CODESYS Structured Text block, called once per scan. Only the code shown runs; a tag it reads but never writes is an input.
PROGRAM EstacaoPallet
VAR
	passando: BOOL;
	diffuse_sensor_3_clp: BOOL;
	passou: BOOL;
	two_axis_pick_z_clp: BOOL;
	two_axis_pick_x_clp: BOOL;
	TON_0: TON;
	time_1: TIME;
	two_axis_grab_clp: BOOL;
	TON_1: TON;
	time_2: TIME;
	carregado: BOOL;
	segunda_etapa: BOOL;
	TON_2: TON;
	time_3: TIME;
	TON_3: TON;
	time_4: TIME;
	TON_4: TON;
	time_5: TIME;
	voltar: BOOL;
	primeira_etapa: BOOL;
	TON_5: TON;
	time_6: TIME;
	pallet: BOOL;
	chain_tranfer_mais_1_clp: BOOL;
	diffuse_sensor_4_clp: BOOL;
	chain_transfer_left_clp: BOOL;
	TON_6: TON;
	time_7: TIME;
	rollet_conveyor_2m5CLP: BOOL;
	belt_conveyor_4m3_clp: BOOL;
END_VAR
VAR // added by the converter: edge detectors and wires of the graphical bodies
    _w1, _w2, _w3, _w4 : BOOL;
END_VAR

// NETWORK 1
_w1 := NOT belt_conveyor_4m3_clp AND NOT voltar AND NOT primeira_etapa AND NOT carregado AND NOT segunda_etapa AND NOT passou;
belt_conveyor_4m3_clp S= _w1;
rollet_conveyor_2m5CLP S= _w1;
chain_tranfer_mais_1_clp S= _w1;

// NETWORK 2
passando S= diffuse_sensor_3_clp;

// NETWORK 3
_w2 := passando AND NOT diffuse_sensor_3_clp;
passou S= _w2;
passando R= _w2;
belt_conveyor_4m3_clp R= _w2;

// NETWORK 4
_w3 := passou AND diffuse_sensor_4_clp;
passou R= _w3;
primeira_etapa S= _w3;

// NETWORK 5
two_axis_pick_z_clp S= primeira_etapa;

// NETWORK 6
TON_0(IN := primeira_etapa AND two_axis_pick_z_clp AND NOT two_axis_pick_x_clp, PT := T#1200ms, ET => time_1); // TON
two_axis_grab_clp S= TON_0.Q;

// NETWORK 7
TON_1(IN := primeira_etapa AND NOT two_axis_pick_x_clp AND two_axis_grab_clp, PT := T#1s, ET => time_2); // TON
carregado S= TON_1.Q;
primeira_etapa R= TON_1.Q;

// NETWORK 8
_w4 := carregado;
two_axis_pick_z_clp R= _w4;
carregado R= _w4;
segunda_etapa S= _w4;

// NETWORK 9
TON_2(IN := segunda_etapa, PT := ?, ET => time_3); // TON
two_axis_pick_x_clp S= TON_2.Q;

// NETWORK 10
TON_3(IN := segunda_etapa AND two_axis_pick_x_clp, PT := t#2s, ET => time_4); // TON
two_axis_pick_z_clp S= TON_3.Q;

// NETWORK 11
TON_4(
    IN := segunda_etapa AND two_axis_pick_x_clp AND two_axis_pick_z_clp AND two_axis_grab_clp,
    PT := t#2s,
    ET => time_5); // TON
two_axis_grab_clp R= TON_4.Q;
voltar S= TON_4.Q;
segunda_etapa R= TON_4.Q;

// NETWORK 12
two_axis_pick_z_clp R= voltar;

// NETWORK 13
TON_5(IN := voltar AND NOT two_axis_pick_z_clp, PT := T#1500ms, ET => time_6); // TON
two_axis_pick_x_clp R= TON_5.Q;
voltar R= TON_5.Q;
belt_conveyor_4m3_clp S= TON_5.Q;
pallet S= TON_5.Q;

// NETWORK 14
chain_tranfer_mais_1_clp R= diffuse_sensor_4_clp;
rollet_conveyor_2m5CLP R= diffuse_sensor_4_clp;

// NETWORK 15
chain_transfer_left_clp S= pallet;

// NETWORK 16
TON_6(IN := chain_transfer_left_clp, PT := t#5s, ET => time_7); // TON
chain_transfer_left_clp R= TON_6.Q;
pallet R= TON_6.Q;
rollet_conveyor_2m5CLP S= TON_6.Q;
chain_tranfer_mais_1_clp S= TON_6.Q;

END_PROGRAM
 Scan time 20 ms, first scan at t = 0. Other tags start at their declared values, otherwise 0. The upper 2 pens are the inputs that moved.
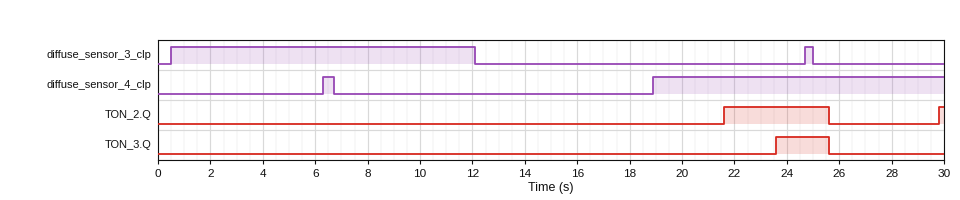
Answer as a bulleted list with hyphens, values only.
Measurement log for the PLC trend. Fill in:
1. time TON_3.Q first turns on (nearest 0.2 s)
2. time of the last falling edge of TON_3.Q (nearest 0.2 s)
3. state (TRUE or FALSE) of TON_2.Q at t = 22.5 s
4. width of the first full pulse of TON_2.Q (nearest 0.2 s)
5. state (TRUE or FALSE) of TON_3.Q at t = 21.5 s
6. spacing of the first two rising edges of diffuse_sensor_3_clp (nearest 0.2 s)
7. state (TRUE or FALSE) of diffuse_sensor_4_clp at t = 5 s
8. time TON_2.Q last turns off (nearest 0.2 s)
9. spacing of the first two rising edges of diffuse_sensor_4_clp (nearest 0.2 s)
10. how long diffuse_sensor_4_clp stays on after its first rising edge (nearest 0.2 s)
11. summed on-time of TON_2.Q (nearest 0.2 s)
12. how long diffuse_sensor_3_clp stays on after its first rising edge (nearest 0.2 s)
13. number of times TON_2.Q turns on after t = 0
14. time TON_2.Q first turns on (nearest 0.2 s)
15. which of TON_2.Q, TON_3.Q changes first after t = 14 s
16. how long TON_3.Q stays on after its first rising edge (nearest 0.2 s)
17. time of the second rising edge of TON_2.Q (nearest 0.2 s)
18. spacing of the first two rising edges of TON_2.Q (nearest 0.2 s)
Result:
- 23.6 s
- 25.6 s
- TRUE
- 4.0 s
- FALSE
- 24.2 s
- FALSE
- 25.6 s
- 12.6 s
- 0.4 s
- 4.2 s
- 11.6 s
- 2
- 21.6 s
- TON_2.Q
- 2.0 s
- 29.8 s
- 8.2 s
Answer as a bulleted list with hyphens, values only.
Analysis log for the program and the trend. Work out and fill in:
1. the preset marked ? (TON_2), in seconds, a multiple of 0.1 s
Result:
- 0.5 s
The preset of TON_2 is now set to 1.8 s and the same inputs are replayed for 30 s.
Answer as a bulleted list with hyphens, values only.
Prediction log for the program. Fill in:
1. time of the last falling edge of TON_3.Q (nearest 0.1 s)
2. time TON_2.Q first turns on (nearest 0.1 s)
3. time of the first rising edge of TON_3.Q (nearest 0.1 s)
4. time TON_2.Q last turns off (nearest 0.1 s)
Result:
- 26.9 s
- 22.9 s
- 24.9 s
- 26.9 s
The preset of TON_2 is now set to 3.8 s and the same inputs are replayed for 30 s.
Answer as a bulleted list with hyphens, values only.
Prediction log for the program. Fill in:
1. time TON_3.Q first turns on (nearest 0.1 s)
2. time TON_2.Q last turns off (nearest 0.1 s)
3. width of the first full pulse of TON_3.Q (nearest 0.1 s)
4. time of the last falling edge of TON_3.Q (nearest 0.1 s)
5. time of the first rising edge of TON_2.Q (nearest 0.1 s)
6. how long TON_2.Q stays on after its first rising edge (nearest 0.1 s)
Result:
- 26.9 s
- 27.0 s
- 0.1 s
- 27.0 s
- 24.9 s
- 2.1 s
